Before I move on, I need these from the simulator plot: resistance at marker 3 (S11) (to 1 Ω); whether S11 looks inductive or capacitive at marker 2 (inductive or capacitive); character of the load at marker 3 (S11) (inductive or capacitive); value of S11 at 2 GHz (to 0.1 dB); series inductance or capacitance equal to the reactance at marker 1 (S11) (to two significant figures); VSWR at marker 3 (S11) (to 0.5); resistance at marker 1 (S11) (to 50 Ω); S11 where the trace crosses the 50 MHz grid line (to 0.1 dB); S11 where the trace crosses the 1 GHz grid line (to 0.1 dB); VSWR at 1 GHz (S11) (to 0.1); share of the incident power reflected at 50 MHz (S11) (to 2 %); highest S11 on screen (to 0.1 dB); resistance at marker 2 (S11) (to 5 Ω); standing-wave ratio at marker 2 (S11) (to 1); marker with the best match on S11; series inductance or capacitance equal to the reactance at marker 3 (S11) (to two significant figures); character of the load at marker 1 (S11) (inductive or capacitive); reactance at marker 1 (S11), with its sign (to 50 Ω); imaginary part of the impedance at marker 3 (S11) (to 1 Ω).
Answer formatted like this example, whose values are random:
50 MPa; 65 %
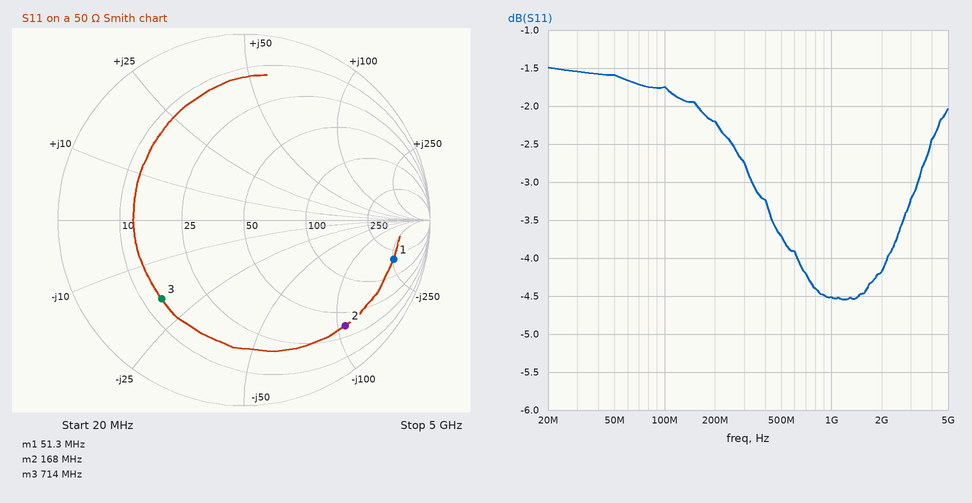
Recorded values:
14 Ω; capacitive; capacitive; -4.2 dB; 12 pF; 4.0; 200 Ω; -1.6 dB; -4.5 dB; 3.9; 70 %; -1.5 dB; 35 Ω; 8; marker 3; 12 pF; capacitive; -250 Ω; -19 Ω
